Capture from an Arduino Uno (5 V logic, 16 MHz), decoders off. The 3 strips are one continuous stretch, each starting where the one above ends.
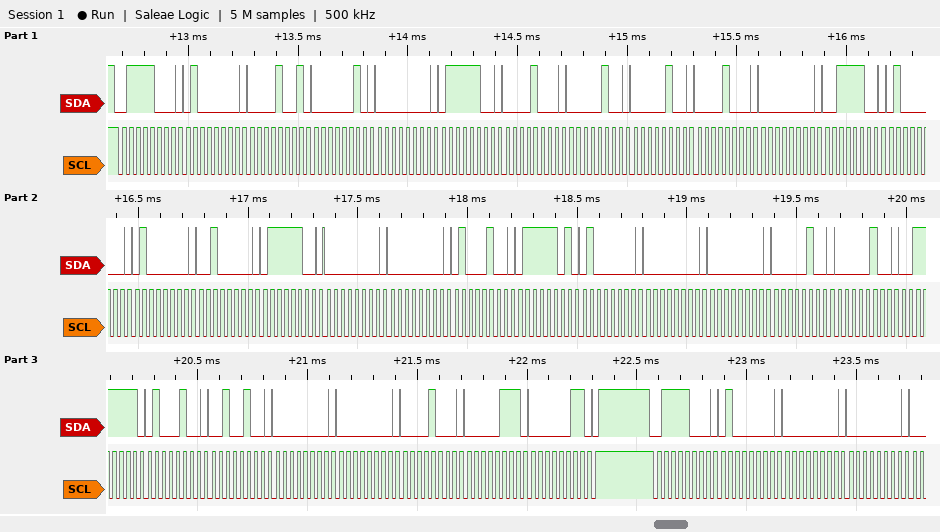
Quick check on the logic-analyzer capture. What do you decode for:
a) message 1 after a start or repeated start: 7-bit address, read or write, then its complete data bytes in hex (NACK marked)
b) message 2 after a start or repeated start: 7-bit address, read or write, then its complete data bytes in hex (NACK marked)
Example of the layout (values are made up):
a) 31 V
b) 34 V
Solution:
a) 0x3C write: 40 09 02 00 7C 08 04 04 08 00 3C 40 40 20 7C 00 00 44 7D 40 00 00 04 04 3F 44 24 00 00 08 07 03
b) 0x3C write: 40 00 00
